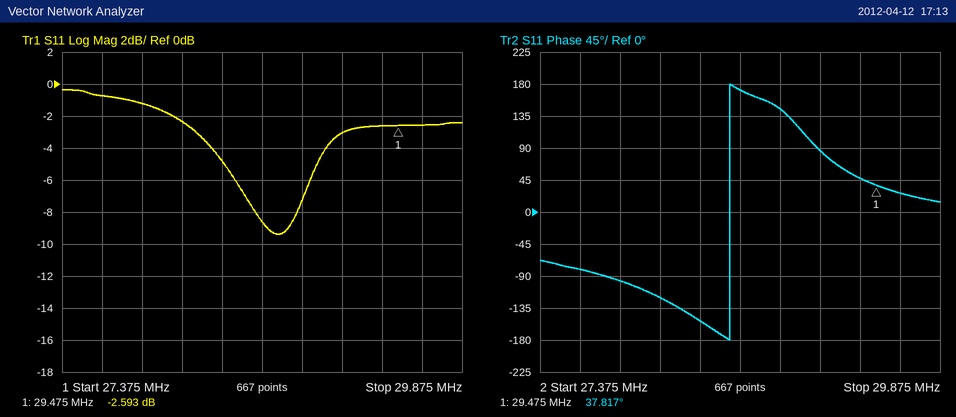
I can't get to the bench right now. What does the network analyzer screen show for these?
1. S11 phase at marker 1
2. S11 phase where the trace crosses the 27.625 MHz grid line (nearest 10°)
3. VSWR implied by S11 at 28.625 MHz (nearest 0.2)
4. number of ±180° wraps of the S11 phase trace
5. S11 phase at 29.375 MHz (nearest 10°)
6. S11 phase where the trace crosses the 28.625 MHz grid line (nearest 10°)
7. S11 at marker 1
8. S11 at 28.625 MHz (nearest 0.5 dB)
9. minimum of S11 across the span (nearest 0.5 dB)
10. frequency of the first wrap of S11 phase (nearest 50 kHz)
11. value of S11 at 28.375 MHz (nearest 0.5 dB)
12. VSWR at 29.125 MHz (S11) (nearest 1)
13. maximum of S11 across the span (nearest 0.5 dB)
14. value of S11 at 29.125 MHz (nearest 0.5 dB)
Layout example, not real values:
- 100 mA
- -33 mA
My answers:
- 37.817°
- -80°
- 2.2
- 1
- 50°
- 170°
- -2.593 dB
- -8.5 dB
- -9.5 dB
- 28.55 MHz
- -5.0 dB
- 6
- -0.5 dB
- -3.0 dB
